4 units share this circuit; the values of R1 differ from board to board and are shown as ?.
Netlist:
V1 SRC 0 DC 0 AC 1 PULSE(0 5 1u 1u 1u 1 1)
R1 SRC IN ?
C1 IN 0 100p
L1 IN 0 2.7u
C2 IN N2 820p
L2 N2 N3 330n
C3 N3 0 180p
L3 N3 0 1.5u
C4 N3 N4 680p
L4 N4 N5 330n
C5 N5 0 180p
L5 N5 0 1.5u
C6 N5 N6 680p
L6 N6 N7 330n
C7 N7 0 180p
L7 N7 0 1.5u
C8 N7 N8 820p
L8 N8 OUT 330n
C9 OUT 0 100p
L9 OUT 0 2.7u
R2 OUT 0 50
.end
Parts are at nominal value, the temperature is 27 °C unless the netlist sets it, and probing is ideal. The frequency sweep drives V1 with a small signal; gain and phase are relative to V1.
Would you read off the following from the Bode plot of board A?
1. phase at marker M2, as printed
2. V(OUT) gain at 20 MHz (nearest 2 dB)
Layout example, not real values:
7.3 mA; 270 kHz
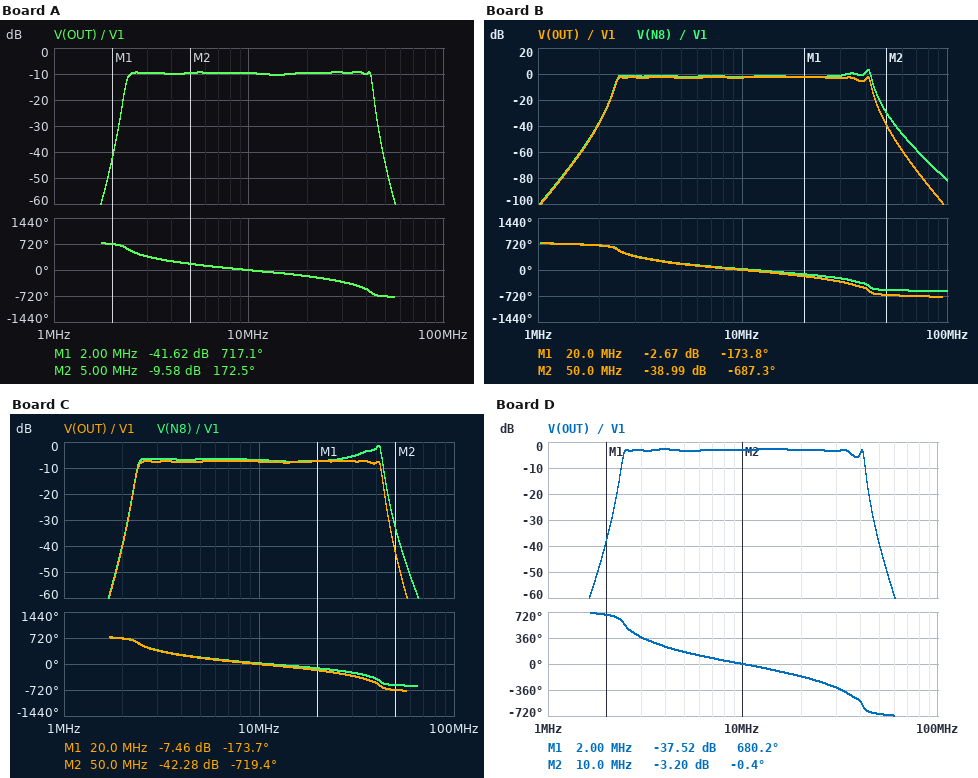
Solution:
172.5 deg; -10 dB
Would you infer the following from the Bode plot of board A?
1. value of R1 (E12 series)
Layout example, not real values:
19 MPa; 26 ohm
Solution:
100 Ω
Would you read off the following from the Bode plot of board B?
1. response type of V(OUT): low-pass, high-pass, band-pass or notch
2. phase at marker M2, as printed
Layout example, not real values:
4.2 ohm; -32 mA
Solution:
band-pass; -687.3 deg
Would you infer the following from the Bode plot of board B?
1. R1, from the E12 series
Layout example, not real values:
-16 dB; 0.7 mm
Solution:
18 Ω
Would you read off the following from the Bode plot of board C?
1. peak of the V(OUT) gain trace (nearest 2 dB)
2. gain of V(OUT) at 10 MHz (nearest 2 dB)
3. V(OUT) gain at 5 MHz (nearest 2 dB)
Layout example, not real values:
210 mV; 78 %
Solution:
-8 dB; -8 dB; -8 dB
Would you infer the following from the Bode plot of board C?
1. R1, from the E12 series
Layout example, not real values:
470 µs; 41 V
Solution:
68 Ω
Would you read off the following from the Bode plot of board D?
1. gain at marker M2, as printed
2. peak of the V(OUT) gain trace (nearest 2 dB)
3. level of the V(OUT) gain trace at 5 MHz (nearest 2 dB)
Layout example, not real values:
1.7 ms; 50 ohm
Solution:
-3.20 dB; -2 dB; -4 dB
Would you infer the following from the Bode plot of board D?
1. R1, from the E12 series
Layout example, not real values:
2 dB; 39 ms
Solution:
22 Ω
